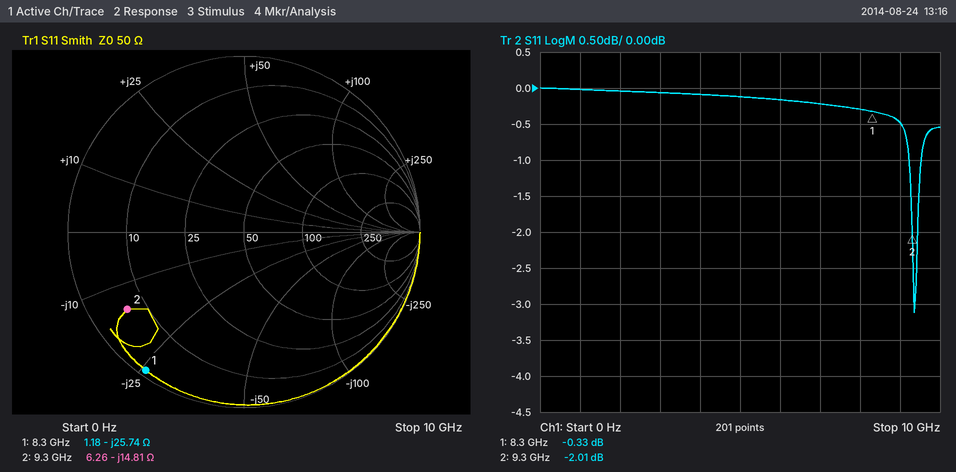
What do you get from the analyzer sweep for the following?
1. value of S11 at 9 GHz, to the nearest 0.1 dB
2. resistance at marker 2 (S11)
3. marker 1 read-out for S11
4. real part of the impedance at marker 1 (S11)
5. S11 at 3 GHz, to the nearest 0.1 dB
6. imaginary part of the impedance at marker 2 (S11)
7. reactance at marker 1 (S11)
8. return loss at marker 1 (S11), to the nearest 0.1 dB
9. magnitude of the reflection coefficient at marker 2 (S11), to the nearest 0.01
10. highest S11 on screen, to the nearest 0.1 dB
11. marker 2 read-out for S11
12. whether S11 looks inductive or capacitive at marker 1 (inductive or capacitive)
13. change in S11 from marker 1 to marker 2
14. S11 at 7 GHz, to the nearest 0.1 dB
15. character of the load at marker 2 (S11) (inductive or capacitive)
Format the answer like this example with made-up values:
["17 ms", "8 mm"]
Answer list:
["-0.5 dB", "6.26 Ω", "-0.33 dB", "1.18 Ω", "-0.1 dB", "-14.81 Ω", "-25.74 Ω", "0.3 dB", "0.79", "0.0 dB", "-2.01 dB", "capacitive", "-1.68 dB", "-0.2 dB", "capacitive"]
